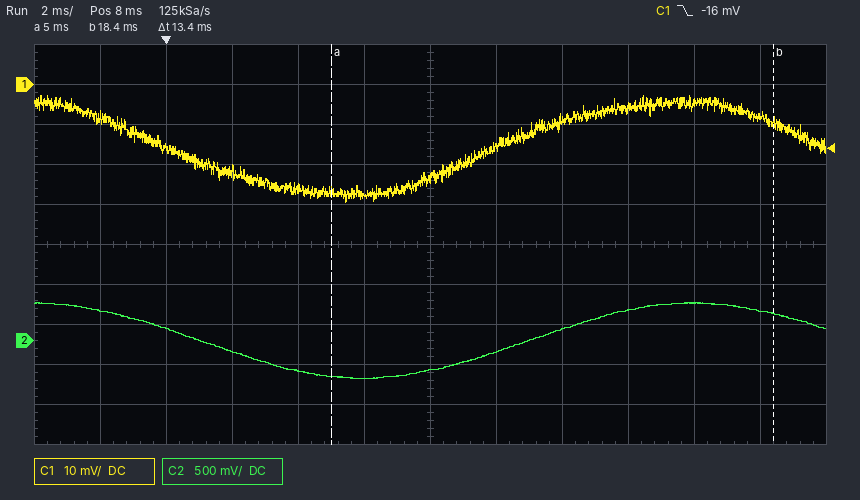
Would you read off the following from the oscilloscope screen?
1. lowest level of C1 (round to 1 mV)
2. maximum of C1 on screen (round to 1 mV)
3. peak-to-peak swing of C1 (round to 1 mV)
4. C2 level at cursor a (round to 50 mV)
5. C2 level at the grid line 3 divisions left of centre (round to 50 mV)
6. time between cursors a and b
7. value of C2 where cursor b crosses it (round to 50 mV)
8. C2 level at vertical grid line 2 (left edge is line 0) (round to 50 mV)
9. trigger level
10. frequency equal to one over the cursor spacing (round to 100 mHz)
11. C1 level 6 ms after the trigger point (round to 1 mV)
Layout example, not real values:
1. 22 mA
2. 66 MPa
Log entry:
1. -30 mV
2. -3 mV
3. 27 mV
4. -450 mV
5. -150 mV
6. 13.4 ms
7. 350 mV
8. 150 mV
9. -16 mV
10. 74.6 Hz
11. -28 mV
